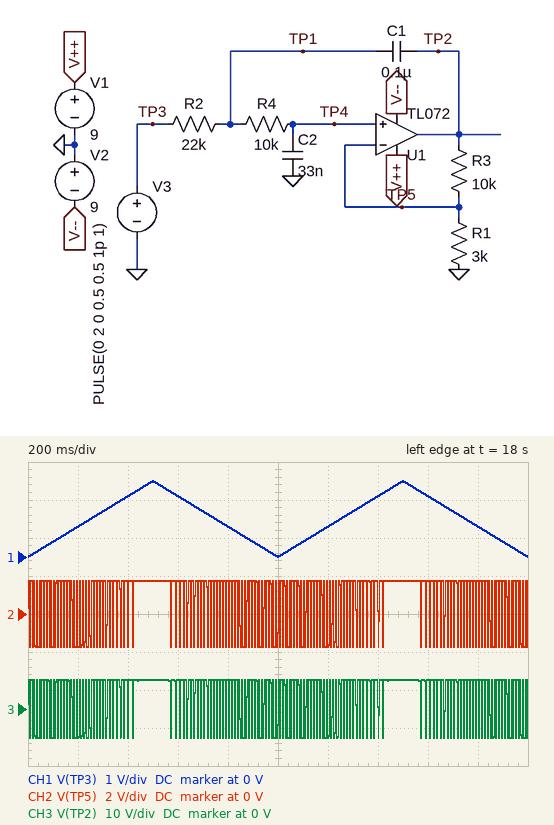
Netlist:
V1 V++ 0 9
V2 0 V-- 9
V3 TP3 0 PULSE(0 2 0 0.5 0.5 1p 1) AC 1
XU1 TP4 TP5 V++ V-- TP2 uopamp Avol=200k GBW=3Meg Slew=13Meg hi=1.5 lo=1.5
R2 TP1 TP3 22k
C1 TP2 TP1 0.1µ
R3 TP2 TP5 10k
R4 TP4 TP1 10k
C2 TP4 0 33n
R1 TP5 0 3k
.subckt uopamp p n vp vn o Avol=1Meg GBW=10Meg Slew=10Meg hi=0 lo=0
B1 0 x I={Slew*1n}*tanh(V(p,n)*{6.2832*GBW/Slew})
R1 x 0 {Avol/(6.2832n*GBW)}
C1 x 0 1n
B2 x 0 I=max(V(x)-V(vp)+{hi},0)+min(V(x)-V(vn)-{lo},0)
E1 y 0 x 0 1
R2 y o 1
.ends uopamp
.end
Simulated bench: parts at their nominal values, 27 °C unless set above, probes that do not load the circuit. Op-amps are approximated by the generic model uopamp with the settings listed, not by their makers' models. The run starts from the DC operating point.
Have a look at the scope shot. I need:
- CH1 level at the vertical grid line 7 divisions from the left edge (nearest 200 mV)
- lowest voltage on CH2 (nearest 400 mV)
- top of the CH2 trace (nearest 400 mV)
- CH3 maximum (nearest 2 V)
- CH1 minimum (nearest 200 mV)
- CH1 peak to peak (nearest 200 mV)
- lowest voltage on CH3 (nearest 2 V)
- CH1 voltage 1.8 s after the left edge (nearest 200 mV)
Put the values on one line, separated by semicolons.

1.6 V; -1.6 V; 1.6 V; 8 V; 0 V; 2.0 V; -8 V; 800 mV
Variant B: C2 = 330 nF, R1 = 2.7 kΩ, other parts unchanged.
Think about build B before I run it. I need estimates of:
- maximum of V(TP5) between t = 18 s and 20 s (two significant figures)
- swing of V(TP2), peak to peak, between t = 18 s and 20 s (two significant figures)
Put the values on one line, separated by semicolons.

1.6 V; 7.5 V
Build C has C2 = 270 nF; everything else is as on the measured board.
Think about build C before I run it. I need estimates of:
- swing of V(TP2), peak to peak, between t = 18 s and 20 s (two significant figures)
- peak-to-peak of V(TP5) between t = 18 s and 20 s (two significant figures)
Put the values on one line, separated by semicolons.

7.5 V; 1.7 V
